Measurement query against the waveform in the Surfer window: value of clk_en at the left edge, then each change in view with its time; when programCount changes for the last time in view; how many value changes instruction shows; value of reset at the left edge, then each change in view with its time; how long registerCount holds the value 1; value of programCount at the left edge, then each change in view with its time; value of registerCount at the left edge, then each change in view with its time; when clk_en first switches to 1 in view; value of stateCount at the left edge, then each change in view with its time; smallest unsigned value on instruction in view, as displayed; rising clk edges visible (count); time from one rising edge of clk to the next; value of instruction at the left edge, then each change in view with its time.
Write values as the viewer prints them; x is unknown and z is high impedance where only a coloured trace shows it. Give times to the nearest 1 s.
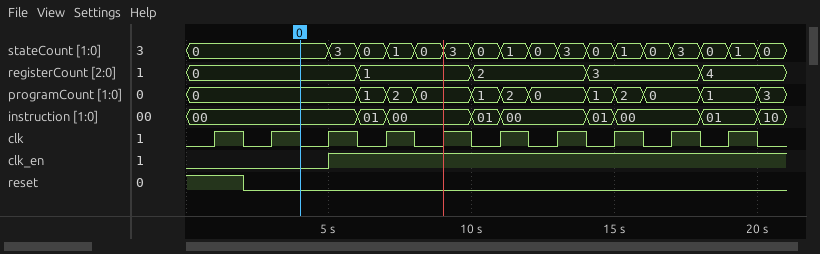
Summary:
0, 1 at 5 s
20 s
8
1, 0 at 2 s
4 s
0, 1 at 6 s, 2 at 7 s, 0 at 8 s, 1 at 10 s, 2 at 11 s, 0 at 12 s, 1 at 14 s, 2 at 15 s, 0 at 16 s, 1 at 18 s, 3 at 20 s
0, 1 at 6 s, 2 at 10 s, 3 at 14 s, 4 at 18 s
5 s
0, 3 at 5 s, 0 at 6 s, 1 at 7 s, 0 at 8 s, 3 at 9 s, 0 at 10 s, 1 at 11 s, 0 at 12 s, 3 at 13 s, 0 at 14 s, 1 at 15 s, 0 at 16 s, 3 at 17 s, 0 at 18 s, 1 at 19 s, 0 at 20 s
00
10
2 s
00, 01 at 6 s, 00 at 7 s, 01 at 10 s, 00 at 11 s, 01 at 14 s, 00 at 15 s, 01 at 18 s, 10 at 20 s
